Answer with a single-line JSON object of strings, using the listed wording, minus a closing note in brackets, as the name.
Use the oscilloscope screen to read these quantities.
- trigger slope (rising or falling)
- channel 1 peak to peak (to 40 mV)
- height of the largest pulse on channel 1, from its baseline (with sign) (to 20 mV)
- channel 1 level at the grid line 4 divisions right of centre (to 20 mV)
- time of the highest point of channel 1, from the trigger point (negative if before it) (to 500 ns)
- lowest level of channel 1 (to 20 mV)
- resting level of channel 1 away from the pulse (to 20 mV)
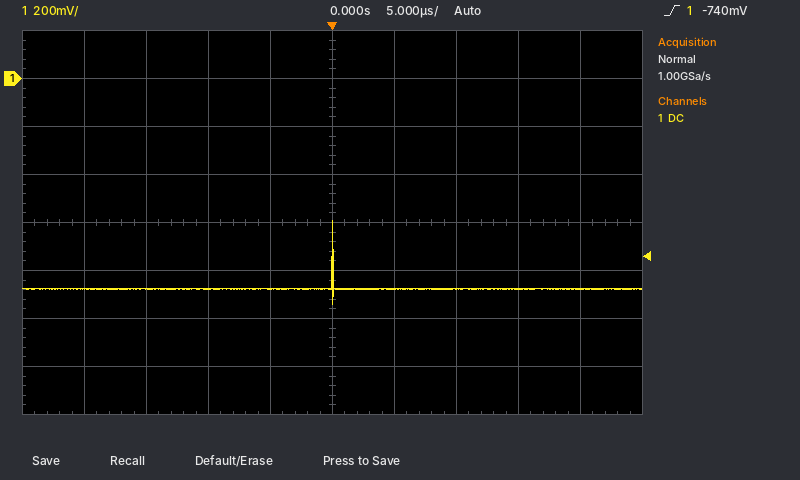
{"trigger slope": "rising", "channel 1 peak to peak": "360 mV", "height of the largest pulse on channel 1, from its baseline (with sign)": "+280 mV", "channel 1 level at the grid line 4 divisions right of centre": "-880 mV", "time of the highest point of channel 1, from the trigger point (negative if before it)": "0.0 µs", "lowest level of channel 1": "-940 mV", "resting level of channel 1 away from the pulse": "-880 mV"}
